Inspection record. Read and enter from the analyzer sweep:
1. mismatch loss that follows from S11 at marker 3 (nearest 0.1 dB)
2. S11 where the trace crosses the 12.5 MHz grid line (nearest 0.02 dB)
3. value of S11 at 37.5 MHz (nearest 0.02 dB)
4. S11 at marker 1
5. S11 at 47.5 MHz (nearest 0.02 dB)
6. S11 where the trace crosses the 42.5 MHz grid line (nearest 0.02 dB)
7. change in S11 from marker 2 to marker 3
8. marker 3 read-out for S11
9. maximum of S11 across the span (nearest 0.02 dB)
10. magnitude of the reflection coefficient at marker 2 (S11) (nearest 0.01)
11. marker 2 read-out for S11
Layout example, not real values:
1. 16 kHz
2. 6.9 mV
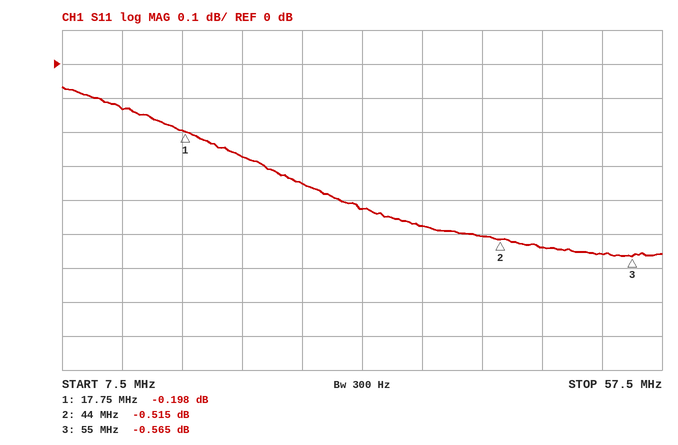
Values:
1. 9.1 dB
2. -0.14 dB
3. -0.48 dB
4. -0.198 dB
5. -0.54 dB
6. -0.50 dB
7. -0.050 dB
8. -0.565 dB
9. -0.06 dB
10. 0.94
11. -0.515 dB
